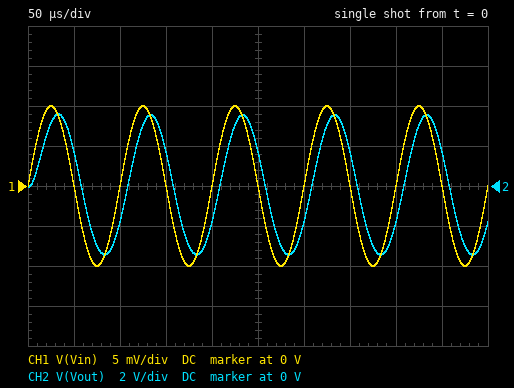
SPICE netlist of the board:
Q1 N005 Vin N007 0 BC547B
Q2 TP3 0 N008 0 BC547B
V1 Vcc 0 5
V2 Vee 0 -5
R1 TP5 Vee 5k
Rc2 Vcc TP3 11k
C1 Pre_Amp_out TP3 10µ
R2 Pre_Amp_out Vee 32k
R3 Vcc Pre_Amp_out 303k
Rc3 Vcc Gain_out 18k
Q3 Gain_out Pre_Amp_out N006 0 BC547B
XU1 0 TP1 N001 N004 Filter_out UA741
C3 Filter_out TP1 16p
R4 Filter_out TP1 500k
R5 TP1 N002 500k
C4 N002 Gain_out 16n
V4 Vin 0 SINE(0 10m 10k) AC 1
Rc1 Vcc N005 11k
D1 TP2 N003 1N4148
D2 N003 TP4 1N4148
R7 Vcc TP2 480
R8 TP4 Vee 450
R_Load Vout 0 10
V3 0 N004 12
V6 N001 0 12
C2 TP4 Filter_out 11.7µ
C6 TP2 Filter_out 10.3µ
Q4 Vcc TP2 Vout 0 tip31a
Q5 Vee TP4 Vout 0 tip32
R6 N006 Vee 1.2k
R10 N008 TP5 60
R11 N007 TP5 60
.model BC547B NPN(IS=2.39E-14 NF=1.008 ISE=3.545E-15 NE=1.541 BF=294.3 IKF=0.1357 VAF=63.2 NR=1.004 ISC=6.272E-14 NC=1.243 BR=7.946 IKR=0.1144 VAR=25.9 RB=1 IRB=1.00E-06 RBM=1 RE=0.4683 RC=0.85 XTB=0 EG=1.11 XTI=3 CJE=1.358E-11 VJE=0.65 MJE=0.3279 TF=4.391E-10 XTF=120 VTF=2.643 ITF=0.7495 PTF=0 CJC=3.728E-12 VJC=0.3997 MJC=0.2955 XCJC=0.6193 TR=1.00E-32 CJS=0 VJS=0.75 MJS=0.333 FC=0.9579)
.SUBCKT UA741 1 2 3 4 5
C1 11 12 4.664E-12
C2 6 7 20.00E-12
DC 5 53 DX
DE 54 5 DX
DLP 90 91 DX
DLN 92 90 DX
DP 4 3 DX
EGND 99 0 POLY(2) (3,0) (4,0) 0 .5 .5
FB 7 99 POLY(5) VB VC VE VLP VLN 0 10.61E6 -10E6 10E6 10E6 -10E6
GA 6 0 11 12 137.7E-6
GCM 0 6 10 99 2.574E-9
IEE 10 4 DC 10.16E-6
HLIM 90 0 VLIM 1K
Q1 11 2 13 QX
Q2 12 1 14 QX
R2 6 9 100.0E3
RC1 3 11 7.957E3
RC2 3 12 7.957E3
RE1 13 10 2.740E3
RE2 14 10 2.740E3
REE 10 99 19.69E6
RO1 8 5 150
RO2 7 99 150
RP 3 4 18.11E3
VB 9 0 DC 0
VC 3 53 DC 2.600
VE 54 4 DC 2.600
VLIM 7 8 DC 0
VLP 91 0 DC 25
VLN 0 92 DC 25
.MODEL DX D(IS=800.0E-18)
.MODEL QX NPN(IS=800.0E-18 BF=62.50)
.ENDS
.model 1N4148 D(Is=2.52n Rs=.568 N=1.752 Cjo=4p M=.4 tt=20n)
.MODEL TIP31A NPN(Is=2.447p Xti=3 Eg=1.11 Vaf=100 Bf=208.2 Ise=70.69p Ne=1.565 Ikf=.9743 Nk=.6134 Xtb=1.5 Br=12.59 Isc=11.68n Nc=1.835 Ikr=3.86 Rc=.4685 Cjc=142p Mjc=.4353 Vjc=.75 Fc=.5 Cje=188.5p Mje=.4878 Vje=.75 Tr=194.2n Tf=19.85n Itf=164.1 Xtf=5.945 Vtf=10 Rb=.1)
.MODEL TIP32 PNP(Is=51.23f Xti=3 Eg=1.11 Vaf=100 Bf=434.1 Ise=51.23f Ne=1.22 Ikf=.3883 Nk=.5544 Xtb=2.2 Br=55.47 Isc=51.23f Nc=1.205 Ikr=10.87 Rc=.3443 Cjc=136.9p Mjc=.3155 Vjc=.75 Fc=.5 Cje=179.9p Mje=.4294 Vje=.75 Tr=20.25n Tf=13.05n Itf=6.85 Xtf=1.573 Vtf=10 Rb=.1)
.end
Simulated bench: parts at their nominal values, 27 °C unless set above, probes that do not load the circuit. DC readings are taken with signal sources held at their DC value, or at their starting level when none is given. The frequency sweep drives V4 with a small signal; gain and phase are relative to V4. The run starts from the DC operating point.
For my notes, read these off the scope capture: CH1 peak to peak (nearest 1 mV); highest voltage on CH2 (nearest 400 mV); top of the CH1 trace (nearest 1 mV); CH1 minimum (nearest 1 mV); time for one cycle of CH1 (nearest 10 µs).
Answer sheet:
20 mV
3.6 V
10 mV
-10 mV
100 µs
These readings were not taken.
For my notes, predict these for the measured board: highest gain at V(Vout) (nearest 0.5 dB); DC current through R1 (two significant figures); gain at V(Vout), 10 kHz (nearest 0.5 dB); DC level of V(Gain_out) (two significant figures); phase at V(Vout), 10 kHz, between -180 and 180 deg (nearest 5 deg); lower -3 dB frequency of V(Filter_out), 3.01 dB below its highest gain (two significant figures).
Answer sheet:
52.0 dB
870 µA
51.0 dB
120 mV
-30 deg
19 Hz
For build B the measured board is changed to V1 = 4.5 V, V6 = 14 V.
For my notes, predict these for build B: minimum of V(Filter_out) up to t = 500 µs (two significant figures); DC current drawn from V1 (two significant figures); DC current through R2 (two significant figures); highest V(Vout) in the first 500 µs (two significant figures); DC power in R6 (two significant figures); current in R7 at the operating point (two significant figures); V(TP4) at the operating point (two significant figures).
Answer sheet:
-2.8 V
85 mA
28 µA
2.6 V
68 µW
8.6 mA
-1.0 V
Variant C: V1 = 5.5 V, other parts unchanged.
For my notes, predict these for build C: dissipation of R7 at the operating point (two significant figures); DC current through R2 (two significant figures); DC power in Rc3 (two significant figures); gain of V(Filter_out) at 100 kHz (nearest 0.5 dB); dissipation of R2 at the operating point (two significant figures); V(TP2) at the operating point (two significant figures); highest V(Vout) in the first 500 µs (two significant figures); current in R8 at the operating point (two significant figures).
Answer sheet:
47 mW
30 µA
1.7 mW
37.5 dB
30 µW
770 mV
3.8 V
9.8 mA
